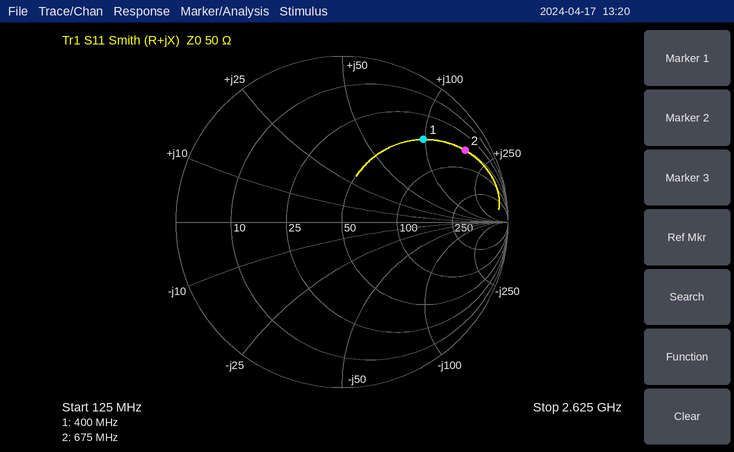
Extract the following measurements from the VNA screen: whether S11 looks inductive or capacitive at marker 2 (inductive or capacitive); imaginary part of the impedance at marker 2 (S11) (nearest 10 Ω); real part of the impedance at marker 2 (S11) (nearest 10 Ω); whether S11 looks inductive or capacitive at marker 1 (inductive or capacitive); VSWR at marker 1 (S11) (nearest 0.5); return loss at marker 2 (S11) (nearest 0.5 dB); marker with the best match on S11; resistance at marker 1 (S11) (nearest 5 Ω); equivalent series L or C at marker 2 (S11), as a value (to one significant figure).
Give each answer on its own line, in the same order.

inductive
+170 Ω
50 Ω
inductive
5.5
1.5 dB
marker 1
50 Ω
40 nH
